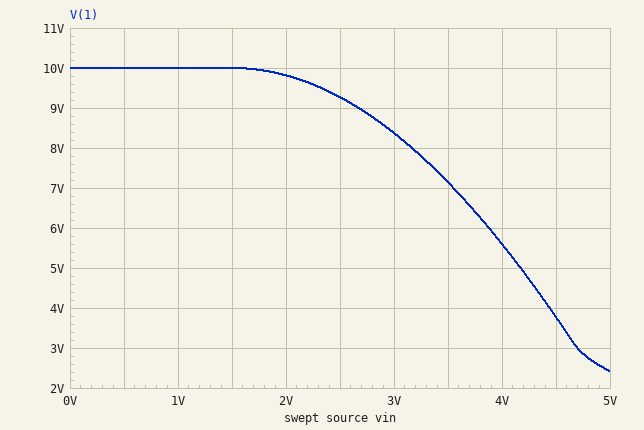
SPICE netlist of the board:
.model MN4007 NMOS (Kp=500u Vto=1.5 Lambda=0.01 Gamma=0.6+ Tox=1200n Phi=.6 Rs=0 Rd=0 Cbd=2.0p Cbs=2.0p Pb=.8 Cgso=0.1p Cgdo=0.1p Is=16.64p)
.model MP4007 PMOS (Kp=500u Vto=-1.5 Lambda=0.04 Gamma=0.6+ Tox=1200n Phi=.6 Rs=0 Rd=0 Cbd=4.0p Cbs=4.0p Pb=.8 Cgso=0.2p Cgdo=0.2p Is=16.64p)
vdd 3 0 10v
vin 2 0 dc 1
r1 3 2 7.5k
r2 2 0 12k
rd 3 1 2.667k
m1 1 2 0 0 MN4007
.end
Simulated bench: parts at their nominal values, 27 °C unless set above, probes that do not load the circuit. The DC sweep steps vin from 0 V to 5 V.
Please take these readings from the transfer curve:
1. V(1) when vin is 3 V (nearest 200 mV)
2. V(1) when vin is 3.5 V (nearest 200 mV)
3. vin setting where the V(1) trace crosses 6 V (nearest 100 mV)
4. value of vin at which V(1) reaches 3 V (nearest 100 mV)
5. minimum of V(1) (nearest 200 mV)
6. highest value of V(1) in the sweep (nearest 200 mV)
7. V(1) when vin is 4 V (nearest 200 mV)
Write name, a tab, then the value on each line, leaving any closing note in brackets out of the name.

V(1) when vin is 3 V	8.4 V
V(1) when vin is 3.5 V	7.2 V
vin setting where the V(1) trace crosses 6 V	3.9 V
value of vin at which V(1) reaches 3 V	4.7 V
minimum of V(1)	2.4 V
highest value of V(1) in the sweep	10.0 V
V(1) when vin is 4 V	5.6 V
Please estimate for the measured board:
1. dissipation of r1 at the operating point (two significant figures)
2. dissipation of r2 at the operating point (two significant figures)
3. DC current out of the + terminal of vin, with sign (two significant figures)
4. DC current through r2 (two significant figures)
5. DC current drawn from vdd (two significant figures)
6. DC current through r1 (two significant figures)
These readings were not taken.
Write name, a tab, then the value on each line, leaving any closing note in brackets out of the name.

dissipation of r1 at the operating point	11 mW
dissipation of r2 at the operating point	83 µW
DC current out of the + terminal of vin, with sign	-1.1 mA
DC current through r2	83 µA
DC current drawn from vdd	1.2 mA
DC current through r1	1.2 mA
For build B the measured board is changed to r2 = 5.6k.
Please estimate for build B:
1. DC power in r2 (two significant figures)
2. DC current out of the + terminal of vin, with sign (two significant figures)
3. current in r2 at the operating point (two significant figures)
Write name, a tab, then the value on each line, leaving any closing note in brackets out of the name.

DC power in r2	180 µW
DC current out of the + terminal of vin, with sign	-1.0 mA
current in r2 at the operating point	180 µA
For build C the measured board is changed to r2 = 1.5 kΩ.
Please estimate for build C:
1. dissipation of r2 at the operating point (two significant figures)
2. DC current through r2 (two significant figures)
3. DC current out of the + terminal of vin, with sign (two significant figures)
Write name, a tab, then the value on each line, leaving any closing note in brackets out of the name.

dissipation of r2 at the operating point	670 µW
DC current through r2	670 µA
DC current out of the + terminal of vin, with sign	-530 µA
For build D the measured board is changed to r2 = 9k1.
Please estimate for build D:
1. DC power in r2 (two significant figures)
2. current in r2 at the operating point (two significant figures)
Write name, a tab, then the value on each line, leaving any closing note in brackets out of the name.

DC power in r2	110 µW
current in r2 at the operating point	110 µA
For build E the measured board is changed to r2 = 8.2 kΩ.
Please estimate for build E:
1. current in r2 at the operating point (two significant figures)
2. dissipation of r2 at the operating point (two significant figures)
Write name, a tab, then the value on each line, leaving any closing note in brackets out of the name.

current in r2 at the operating point	120 µA
dissipation of r2 at the operating point	120 µW
